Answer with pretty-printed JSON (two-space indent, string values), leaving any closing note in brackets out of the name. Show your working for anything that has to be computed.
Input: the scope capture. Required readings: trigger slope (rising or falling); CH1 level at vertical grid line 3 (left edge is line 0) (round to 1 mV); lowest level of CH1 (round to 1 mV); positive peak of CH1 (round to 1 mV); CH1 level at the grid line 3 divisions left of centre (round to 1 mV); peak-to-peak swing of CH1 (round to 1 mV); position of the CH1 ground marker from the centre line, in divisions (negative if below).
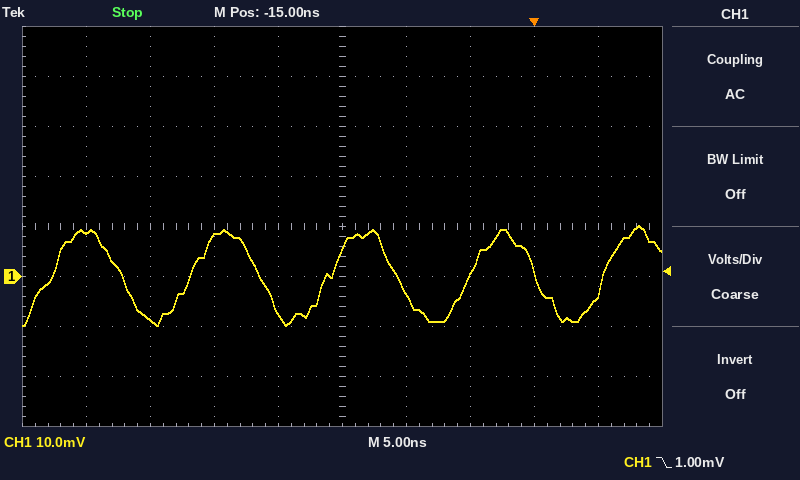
{
  "trigger slope": "falling",
  "CH1 level at vertical grid line 3 (left edge is line 0)": "8 mV",
  "lowest level of CH1": "-10 mV",
  "positive peak of CH1": "10 mV",
  "CH1 level at the grid line 3 divisions left of centre": "-9 mV",
  "peak-to-peak swing of CH1": "10 mV − (-10 mV) = 20 mV",
  "position of the CH1 ground marker from the centre line, in divisions": "-1.0 div"
}
